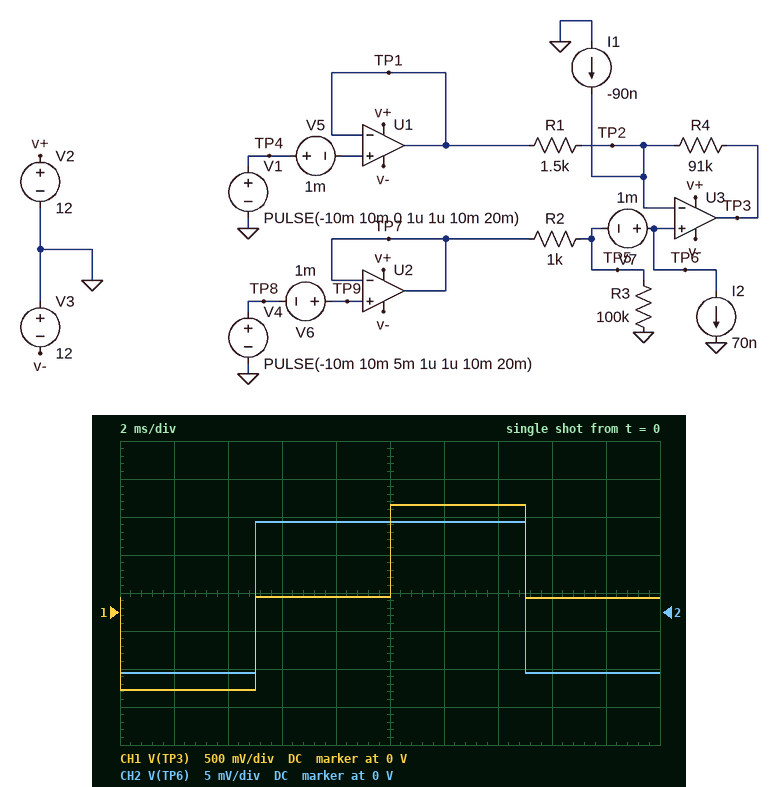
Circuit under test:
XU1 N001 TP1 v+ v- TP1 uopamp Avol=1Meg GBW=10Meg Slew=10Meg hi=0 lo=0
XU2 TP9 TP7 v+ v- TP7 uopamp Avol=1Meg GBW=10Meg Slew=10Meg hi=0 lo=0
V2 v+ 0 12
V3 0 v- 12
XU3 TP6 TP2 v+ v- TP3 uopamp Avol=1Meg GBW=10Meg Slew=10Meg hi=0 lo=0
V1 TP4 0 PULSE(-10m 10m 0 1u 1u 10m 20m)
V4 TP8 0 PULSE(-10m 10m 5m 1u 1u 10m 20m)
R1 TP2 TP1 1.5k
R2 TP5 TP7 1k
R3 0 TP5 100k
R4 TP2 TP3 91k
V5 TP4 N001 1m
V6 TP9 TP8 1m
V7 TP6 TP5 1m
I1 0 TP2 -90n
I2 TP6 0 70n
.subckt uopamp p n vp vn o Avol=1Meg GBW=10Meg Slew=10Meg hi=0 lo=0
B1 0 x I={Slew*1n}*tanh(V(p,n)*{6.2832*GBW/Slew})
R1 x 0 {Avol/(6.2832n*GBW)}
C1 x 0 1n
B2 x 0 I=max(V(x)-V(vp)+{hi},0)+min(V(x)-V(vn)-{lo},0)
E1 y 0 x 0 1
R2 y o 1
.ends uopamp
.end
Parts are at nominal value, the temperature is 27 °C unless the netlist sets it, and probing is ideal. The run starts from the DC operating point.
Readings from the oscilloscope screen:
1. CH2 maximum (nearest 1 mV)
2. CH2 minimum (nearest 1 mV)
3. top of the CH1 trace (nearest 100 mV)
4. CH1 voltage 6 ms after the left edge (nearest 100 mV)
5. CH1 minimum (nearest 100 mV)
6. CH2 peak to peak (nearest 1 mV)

12 mV
-8 mV
1.4 V
200 mV
-1.0 V
20 mV
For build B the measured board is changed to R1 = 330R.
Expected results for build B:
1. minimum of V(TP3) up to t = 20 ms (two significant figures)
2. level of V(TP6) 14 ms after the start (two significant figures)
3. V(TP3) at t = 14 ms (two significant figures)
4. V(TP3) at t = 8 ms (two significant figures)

-4.7 V
12 mV
6.3 V
800 mV
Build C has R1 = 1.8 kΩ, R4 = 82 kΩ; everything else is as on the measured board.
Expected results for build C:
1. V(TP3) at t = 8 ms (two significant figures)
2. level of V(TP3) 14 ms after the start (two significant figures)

150 mV
1.1 V
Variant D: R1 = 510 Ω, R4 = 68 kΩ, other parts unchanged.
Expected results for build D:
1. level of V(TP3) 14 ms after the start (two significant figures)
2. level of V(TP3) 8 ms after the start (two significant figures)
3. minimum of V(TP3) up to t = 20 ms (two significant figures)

3.1 V
390 mV
-2.3 V
